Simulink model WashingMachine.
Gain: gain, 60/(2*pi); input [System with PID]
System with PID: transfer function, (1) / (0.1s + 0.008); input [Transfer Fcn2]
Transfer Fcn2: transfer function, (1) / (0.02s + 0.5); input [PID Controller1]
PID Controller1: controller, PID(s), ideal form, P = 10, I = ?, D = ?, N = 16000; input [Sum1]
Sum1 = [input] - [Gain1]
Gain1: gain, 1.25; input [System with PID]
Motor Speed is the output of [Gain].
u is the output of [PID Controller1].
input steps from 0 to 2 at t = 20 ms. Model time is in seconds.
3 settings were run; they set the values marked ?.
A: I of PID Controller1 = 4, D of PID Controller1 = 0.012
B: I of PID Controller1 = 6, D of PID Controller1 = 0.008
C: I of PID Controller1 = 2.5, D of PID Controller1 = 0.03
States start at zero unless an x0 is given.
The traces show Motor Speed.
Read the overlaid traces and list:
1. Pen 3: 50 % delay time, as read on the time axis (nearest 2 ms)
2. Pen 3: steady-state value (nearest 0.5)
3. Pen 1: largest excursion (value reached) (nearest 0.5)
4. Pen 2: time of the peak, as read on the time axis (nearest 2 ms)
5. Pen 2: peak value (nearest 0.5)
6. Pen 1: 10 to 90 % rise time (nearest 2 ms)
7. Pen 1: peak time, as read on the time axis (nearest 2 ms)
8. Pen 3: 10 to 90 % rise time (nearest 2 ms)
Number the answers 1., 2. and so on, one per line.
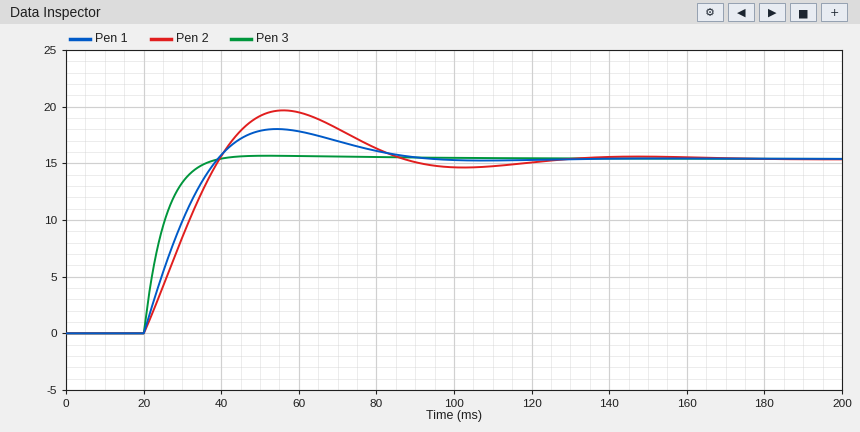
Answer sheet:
1. 24 ms
2. 15.5
3. 18.0
4. 56 ms
5. 19.5
6. 14 ms
7. 54 ms
8. 10 ms
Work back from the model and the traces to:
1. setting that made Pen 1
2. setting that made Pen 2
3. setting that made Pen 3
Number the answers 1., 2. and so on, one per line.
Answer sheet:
1. A
2. B
3. C
